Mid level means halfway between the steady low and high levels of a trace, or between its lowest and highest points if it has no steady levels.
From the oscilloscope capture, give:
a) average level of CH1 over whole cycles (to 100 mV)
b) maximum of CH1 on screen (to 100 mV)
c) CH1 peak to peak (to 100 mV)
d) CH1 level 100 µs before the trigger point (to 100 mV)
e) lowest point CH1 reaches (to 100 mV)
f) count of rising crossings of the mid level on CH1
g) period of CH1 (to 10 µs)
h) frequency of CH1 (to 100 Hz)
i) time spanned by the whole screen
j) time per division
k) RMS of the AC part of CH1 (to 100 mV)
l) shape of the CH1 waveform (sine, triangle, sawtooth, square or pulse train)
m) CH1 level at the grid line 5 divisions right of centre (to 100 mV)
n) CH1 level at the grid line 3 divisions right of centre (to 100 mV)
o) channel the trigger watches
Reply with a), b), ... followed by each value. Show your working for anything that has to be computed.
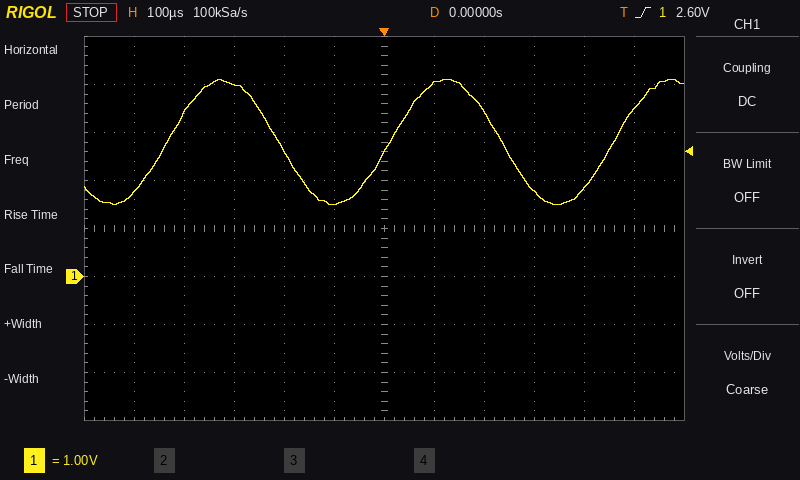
a) (4.1 V + (1.5 V)) / 2 ≈ 2.8 V
b) 4.1 V
c) 4.1 V − (1.5 V) = 2.6 V
d) 1.5 V
e) 1.5 V
f) 3
g) 450 µs
h) 1 / 450 µs ≈ 2.2 kHz
i) 1.2 ms
j) 100 µs
k) 2.6 V / (2√2) ≈ 919 mV, so 900 mV to the nearest 100 mV
l) sine
m) 3.5 V
n) 1.8 V
o) CH1
